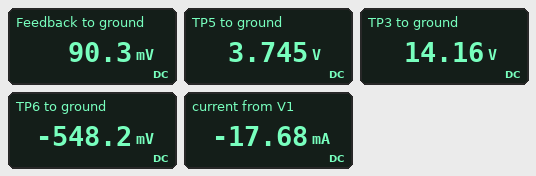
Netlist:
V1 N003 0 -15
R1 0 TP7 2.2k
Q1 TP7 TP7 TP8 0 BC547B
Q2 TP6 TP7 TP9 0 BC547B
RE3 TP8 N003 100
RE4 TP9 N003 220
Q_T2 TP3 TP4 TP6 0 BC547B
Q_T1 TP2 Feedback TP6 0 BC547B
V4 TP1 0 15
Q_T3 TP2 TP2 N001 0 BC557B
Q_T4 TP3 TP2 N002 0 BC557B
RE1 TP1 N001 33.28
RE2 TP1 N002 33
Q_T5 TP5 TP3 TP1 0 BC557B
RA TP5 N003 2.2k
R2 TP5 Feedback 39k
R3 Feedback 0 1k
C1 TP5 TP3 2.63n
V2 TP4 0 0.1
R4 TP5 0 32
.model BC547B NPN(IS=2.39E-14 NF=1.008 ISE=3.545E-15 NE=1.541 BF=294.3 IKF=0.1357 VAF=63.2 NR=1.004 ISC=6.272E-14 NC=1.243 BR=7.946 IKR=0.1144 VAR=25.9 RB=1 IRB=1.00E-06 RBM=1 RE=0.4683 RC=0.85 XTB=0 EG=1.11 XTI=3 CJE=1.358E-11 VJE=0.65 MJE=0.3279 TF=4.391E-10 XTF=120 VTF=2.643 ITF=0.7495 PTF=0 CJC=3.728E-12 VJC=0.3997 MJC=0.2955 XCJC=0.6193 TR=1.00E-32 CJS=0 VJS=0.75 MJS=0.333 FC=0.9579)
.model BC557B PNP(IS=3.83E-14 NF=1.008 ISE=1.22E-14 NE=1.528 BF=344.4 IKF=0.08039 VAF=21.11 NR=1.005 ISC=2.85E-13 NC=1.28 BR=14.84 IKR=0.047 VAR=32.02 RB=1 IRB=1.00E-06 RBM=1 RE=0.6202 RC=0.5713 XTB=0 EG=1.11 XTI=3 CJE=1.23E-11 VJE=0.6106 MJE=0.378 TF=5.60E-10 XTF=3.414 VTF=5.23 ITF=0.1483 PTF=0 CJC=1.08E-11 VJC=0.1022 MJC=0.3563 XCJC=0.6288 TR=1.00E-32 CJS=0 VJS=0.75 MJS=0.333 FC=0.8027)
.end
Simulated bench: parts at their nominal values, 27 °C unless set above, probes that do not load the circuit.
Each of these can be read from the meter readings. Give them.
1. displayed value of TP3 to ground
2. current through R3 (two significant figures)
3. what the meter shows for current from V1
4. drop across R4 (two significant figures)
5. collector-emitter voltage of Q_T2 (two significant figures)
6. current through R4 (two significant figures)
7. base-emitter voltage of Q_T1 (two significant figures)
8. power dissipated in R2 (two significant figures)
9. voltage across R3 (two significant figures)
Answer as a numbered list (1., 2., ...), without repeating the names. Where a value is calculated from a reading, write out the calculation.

1. 14.16 V
2. (90.3 mV) / 1 kΩ = 90 µA
3. -17.68 mA
4. 3.745 V = 3.7 V
5. 14.16 V - (-548.2 mV) = 15 V
6. (3.745 V) / 32 Ω = 120 mA
7. 90.3 mV - (-548.2 mV) = 640 mV
8. (3.745 V - 90.3 mV)^2 / 39 kΩ = 340 µW
9. 90.3 mV = 90 mV
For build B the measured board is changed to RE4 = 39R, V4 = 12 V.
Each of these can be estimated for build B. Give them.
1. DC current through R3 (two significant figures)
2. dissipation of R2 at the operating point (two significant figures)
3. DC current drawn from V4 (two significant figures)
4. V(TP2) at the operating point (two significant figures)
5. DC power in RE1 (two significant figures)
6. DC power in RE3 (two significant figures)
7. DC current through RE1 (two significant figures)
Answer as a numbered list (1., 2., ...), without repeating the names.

1. 96 µA
2. 550 µW
3. 170 mA
4. 11 V
5. 1.7 mW
6. 3.8 mW
7. 7.1 mA
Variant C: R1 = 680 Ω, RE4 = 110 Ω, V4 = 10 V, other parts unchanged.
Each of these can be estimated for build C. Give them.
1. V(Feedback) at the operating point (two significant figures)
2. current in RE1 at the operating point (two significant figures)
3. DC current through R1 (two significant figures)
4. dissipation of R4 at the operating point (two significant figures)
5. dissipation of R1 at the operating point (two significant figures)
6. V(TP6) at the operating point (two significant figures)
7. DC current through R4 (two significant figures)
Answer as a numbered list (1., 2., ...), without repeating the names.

1. 96 mV
2. 7.7 mA
3. 18 mA
4. 720 mW
5. 230 mW
6. -600 mV
7. 150 mA
